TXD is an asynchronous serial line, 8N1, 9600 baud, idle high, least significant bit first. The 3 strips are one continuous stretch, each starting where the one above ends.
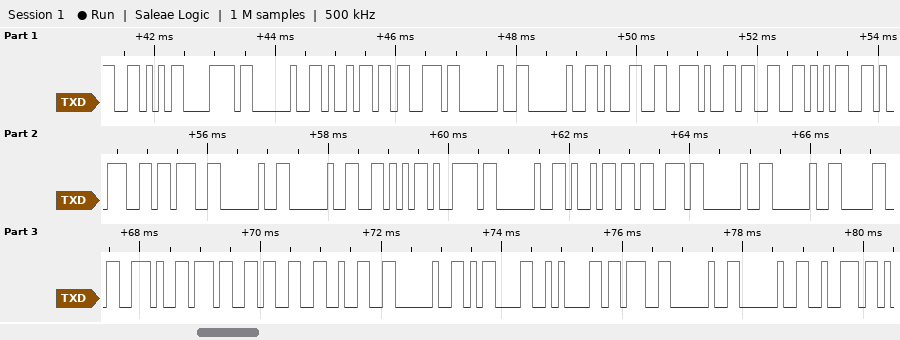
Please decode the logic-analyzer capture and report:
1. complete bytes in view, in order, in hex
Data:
56 78 20 69 73 20 20 31 2E 33 35 39 3B 20 20 56 79 20 69 73 20 20 30 2E 37 33 32 20 0D 0A 3B 20 20 72
